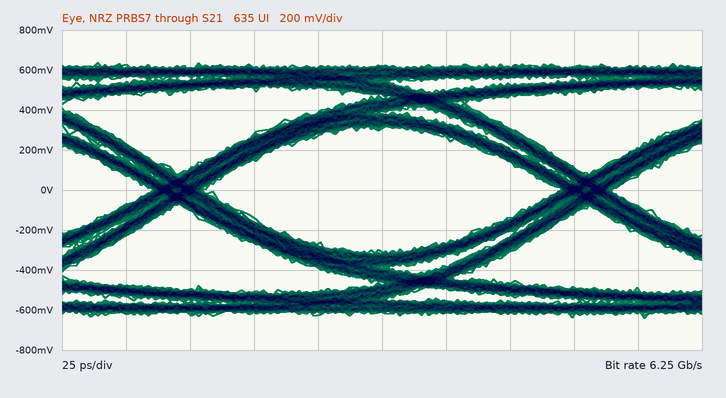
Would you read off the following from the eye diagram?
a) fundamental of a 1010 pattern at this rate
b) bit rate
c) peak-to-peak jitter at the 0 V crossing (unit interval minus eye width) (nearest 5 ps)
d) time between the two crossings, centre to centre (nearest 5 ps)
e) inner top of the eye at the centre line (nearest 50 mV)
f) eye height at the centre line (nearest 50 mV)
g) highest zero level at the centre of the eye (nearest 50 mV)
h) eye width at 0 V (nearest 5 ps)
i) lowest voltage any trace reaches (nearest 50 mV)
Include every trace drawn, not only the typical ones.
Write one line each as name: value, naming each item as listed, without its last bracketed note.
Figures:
fundamental of a 1010 pattern at this rate: 3.125 GHz
bit rate: 6.25 Gb/s
peak-to-peak jitter at the 0 V crossing (unit interval minus eye width): 20 ps
time between the two crossings, centre to centre: 160 ps
inner top of the eye at the centre line: 300 mV
eye height at the centre line: 600 mV
highest zero level at the centre of the eye: -300 mV
eye width at 0 V: 140 ps
lowest voltage any trace reaches: -650 mV
